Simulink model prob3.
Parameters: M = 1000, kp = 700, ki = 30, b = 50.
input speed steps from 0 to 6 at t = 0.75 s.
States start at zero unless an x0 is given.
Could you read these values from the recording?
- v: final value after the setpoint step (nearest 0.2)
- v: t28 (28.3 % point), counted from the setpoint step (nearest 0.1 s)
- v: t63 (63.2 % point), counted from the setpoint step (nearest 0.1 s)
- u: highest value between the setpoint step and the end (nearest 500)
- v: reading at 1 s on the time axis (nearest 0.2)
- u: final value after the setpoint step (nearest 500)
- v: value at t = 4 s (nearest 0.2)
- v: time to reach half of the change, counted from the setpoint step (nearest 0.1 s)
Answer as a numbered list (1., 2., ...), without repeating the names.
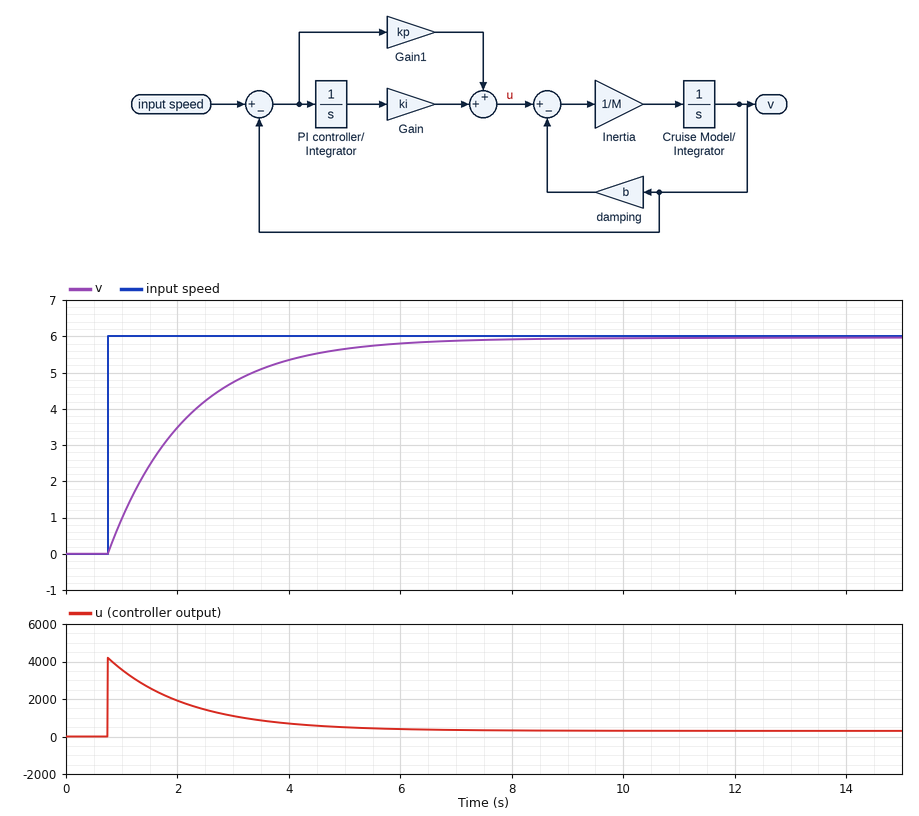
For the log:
1. 6.0
2. 0.5 s
3. 1.4 s
4. 4000
5. 1.0
6. 500
7. 5.4
8. 1.0 s
